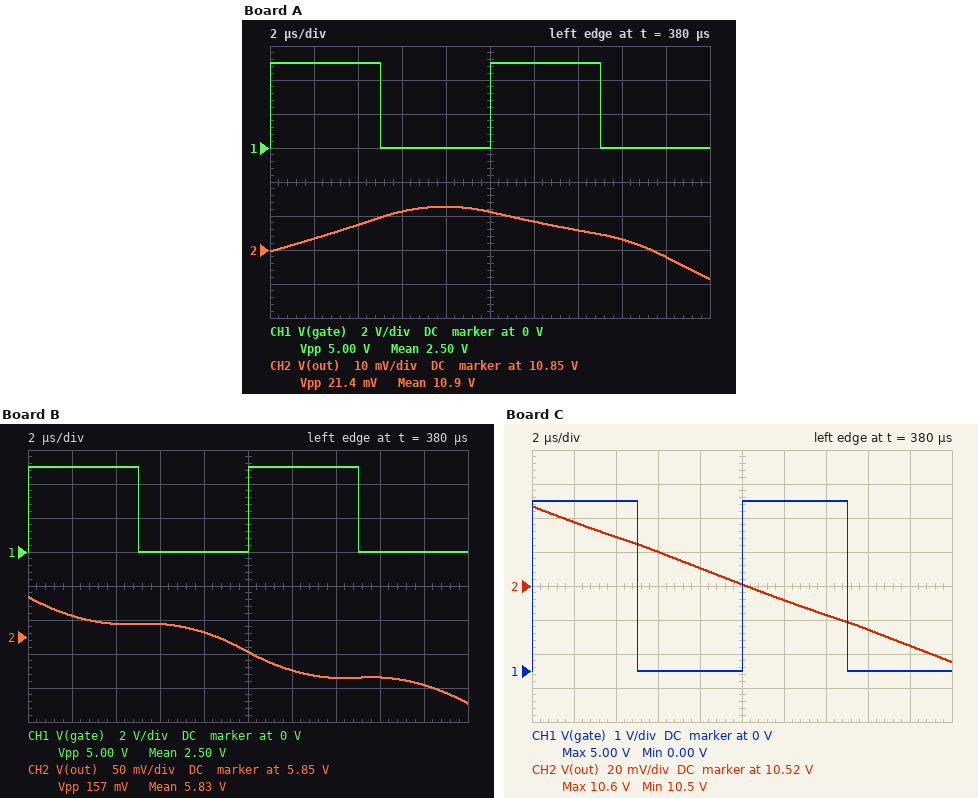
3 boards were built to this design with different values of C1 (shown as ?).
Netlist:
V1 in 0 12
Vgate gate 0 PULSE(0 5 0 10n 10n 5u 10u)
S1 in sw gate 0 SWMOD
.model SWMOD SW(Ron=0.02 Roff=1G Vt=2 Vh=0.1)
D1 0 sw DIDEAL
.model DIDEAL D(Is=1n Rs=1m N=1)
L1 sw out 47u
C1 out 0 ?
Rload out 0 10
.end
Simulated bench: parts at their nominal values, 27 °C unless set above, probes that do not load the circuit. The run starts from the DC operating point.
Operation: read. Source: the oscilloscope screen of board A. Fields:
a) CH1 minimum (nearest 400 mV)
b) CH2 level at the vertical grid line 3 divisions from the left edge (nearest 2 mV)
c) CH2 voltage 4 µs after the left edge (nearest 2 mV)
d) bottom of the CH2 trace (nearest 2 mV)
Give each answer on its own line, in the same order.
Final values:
0 V
10.862 V
10.858 V
10.842 V
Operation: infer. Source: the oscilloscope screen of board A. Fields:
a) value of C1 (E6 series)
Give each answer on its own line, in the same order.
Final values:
330 µF
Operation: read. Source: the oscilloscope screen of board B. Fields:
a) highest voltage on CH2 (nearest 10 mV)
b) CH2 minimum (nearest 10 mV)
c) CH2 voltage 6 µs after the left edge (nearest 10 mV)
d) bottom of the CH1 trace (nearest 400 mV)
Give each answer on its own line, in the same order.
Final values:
5.91 V
5.75 V
5.87 V
0 V
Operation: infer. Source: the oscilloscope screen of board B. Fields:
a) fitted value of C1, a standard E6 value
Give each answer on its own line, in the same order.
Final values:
33 µF
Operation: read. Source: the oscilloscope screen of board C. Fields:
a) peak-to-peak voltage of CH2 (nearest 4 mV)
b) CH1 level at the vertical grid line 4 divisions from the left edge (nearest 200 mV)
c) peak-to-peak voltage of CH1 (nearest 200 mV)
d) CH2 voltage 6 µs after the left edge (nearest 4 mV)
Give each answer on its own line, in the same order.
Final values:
92 mV
0 V
5.0 V
10.540 V
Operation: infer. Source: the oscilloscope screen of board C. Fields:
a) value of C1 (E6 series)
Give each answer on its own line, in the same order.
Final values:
220 µF
